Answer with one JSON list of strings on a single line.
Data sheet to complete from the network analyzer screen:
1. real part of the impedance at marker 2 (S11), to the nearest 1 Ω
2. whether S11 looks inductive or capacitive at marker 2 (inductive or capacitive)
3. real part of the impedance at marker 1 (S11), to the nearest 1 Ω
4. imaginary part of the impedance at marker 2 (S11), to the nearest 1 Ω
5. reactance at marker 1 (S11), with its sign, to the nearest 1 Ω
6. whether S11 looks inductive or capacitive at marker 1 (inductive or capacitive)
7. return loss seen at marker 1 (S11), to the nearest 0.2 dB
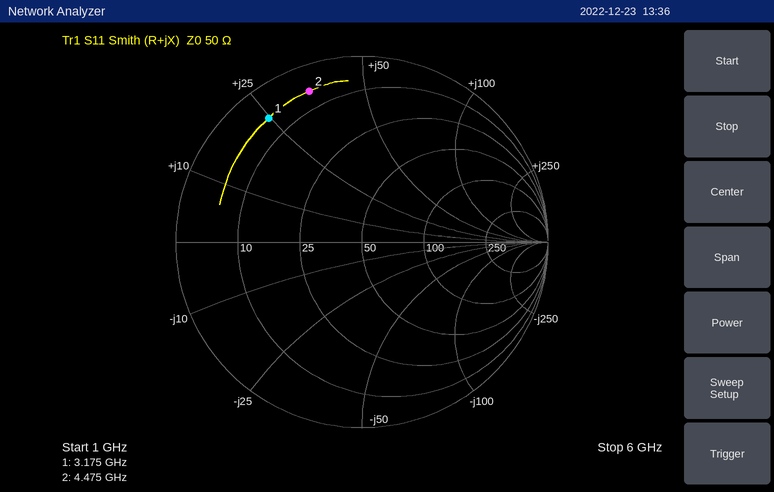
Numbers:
["6 Ω", "inductive", "6 Ω", "+35 Ω", "+25 Ω", "inductive", "1.6 dB"]
